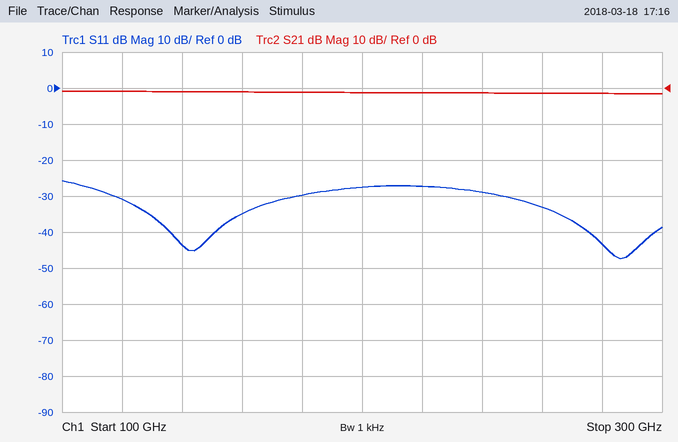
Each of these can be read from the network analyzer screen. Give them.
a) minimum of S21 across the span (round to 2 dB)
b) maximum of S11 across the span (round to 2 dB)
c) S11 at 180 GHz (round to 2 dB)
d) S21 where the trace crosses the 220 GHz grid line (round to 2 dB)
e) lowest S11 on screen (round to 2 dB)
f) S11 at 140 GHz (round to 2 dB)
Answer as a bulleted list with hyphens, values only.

- -2 dB
- -26 dB
- -30 dB
- -2 dB
- -48 dB
- -44 dB
